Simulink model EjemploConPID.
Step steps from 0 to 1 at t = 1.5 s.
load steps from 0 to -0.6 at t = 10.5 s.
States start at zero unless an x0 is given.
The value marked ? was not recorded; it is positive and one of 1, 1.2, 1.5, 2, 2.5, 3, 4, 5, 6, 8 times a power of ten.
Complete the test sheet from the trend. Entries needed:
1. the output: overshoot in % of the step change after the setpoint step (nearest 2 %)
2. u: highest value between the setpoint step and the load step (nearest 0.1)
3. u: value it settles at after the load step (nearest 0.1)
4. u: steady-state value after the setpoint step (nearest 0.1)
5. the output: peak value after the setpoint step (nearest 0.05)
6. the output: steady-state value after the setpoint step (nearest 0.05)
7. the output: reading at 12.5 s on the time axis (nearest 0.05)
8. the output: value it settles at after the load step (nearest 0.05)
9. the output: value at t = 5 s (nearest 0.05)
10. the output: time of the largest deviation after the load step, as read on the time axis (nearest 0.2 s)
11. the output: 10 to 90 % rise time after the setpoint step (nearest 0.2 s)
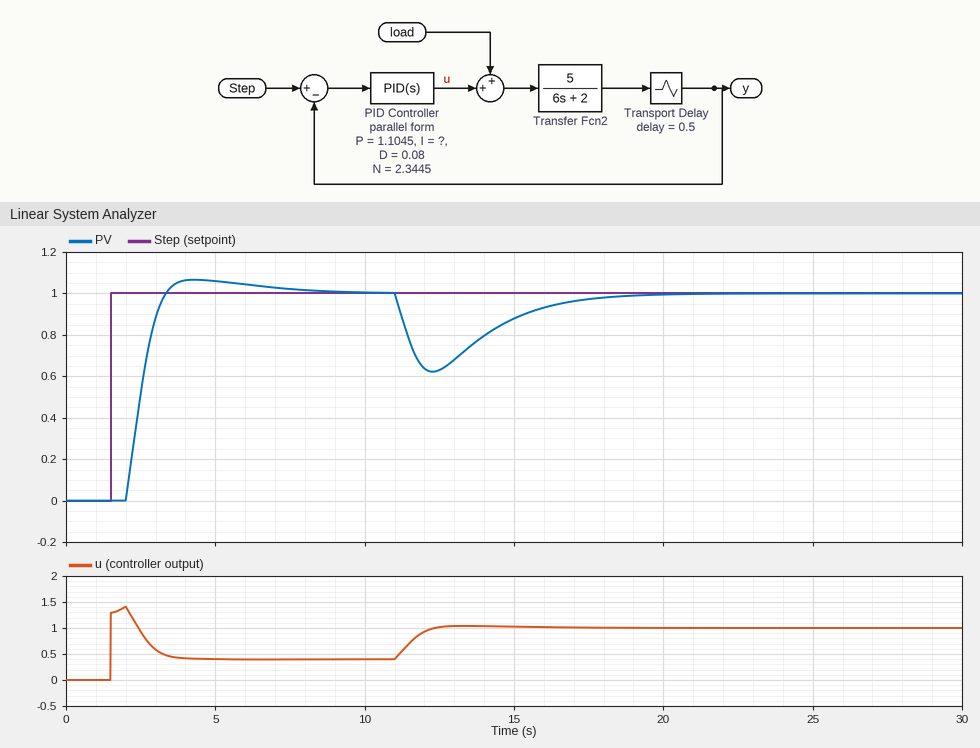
6 %
1.4
1.0
0.4
1.05
1.00
0.65
1.00
1.05
12.2 s
1.0 s
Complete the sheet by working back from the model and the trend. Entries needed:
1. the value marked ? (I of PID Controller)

0.5
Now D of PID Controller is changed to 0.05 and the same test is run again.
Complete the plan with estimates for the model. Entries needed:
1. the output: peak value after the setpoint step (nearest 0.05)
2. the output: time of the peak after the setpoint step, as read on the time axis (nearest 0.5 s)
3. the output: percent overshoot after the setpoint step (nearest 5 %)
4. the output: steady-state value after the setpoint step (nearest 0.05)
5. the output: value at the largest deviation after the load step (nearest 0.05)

1.10
4.0 s
10 %
1.00
0.60
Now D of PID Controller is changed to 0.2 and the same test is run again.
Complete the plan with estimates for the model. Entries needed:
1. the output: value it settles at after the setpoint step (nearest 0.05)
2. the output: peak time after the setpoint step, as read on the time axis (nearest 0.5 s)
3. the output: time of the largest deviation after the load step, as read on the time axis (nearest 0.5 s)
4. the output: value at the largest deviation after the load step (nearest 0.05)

1.00
5.5 s
12.0 s
0.65
